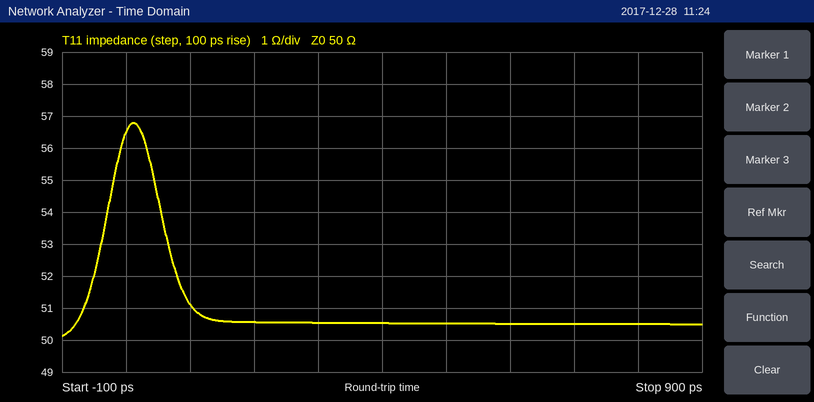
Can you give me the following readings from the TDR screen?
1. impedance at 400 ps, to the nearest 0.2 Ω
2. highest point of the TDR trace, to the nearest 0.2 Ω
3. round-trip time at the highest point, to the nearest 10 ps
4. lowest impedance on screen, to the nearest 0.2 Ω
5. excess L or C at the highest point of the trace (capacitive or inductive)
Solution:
50.6 Ω
56.8 Ω
10 ps
50.2 Ω
inductive
